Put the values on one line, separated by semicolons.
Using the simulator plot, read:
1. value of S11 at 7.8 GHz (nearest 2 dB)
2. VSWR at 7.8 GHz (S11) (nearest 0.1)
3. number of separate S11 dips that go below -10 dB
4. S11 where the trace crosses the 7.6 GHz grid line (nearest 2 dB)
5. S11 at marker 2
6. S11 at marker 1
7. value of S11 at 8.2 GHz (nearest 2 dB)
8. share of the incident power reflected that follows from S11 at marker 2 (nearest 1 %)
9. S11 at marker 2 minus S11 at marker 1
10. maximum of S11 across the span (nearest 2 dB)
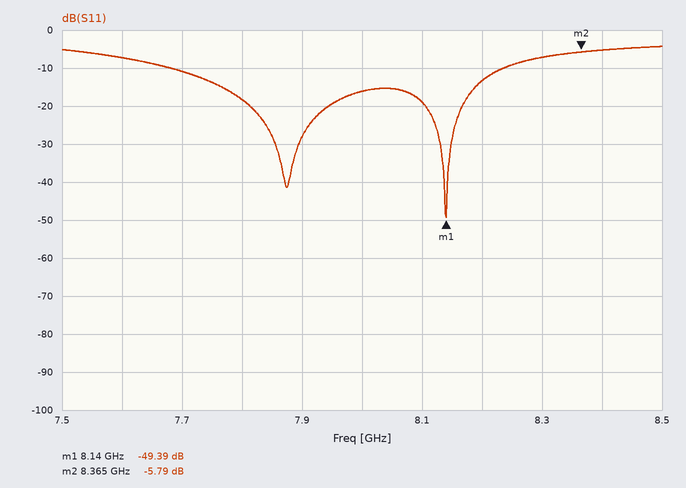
-18 dB; 1.3; 2; -8 dB; -5.79 dB; -49.39 dB; -14 dB; 26 %; 43.60 dB; -4 dB
